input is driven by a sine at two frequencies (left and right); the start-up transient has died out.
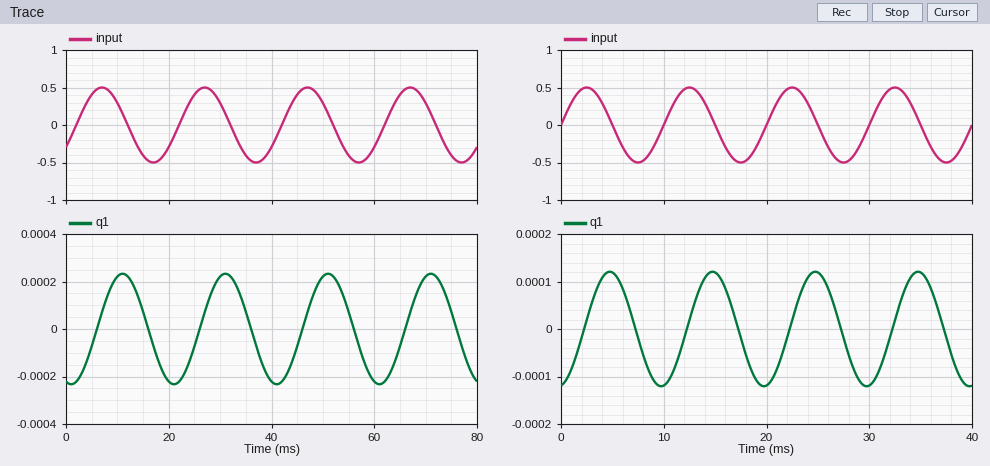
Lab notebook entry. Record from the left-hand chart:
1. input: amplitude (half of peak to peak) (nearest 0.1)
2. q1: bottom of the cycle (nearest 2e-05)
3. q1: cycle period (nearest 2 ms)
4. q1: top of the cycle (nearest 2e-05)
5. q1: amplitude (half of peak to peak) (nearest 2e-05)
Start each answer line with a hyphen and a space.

- 0.5
- -0.00024
- 20 ms
- 0.00024
- 0.00024
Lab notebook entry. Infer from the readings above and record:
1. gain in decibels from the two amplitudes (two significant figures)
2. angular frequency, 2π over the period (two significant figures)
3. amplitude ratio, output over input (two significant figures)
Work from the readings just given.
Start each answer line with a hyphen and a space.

- -66 dB
- 0.31 rad/ms
- 0.00048
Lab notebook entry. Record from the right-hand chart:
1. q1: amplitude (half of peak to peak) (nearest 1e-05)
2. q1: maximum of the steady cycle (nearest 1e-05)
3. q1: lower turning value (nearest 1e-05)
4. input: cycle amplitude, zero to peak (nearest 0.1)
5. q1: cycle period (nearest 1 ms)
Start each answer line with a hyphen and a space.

- 0.00012
- 0.00012
- -0.00012
- 0.5
- 10 ms
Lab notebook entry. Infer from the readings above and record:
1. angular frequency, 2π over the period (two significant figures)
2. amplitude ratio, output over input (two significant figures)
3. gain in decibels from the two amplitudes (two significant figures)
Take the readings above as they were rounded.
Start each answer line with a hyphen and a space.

- 0.63 rad/ms
- 0.00024
- -72 dB
